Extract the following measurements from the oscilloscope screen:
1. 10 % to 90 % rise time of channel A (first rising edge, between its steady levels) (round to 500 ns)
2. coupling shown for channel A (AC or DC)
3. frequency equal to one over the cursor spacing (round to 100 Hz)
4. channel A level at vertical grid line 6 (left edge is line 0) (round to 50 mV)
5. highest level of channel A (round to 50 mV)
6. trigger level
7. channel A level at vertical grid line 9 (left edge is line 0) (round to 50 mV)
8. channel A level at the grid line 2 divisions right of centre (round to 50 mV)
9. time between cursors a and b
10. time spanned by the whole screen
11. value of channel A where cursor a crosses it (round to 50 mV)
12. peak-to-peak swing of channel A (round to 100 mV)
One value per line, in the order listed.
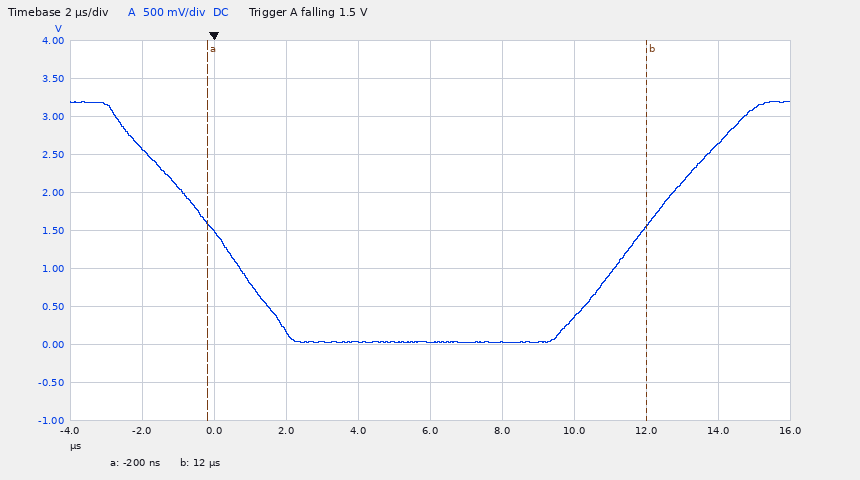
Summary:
4.5 µs
DC
82.0 kHz
50 mV
3.20 V
1.5 V
2.65 V
350 mV
12.2 µs
20 µs
1.60 V
3.20 V
